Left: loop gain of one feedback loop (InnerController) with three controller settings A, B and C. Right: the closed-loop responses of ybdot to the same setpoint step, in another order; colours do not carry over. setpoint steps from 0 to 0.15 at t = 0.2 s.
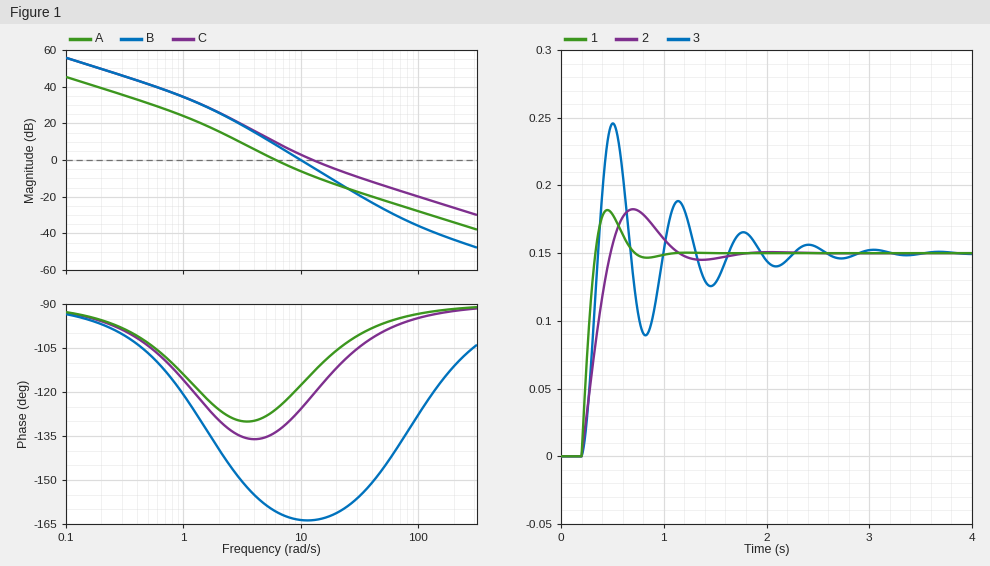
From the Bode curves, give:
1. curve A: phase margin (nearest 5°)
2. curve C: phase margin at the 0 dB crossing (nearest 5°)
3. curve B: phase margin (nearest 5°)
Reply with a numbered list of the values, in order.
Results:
1. 55°
2. 60°
3. 15°
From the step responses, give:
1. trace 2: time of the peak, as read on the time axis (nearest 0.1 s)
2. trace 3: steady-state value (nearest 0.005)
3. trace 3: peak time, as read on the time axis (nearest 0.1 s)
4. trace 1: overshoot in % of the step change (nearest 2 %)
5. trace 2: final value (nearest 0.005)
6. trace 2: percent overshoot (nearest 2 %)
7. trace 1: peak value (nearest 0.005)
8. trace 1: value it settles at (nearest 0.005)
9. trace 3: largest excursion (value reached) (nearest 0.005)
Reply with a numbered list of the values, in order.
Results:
1. 0.7 s
2. 0.150
3. 0.5 s
4. 22 %
5. 0.150
6. 22 %
7. 0.180
8. 0.150
9. 0.245
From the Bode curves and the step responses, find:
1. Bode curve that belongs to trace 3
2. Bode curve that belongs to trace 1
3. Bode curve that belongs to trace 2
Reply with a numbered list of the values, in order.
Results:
1. B
2. C
3. A
